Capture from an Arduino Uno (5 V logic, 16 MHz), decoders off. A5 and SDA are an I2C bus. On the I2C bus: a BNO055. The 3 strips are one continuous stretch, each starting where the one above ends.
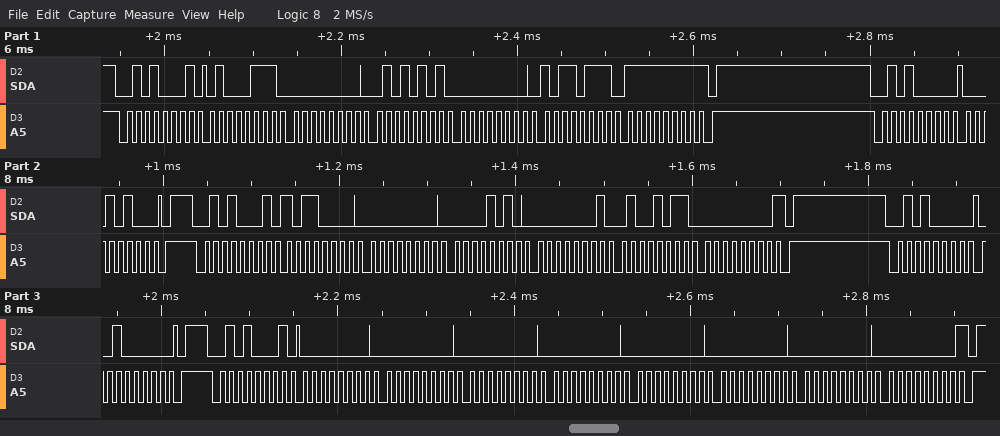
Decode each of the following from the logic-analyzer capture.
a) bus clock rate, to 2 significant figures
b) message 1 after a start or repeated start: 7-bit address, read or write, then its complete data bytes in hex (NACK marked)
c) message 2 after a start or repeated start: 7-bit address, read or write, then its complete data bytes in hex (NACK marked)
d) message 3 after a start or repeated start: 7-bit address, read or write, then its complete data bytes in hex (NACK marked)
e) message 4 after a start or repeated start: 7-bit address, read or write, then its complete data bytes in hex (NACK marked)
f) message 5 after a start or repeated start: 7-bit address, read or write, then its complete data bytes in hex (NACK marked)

100 kHz
0x28 read: 47 00 55 00 B7 FF NACK
0x28 write: 14
0x28 read: B0 00 0A 01 4B 00 NACK
0x28 write: 20
0x28 read: 00 00 00 00 00 00 00 00 NACK
